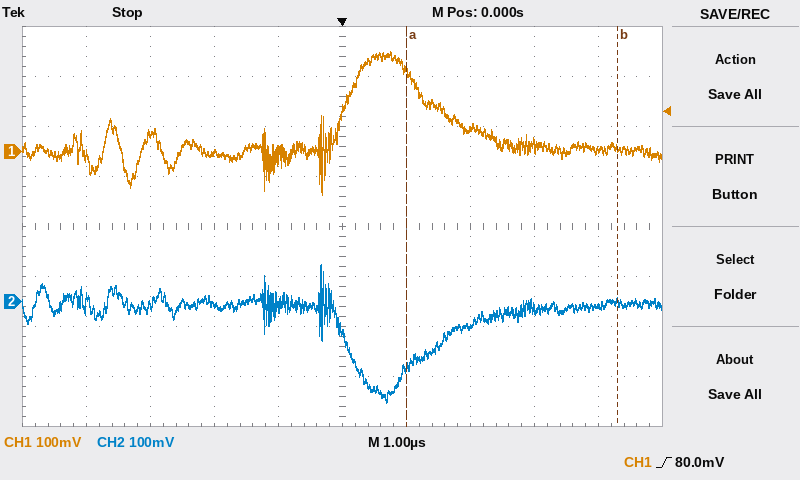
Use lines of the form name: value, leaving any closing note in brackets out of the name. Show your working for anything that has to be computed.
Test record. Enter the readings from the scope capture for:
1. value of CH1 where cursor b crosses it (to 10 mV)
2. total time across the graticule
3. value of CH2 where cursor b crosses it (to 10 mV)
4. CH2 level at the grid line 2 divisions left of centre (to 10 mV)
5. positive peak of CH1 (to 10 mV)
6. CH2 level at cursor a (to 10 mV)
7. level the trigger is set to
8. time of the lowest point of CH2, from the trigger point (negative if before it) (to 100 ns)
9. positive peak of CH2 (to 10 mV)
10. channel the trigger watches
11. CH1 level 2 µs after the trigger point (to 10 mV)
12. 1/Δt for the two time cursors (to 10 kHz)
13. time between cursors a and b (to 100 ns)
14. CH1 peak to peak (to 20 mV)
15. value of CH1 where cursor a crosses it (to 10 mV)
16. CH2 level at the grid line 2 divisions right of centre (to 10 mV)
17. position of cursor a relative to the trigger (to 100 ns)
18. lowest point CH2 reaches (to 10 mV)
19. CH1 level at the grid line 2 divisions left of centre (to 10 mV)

value of CH1 where cursor b crosses it: 10 mV
total time across the graticule: 10 µs
value of CH2 where cursor b crosses it: 0 mV
CH2 level at the grid line 2 divisions left of centre: -10 mV
positive peak of CH1: 200 mV
CH2 level at cursor a: -130 mV
level the trigger is set to: 80.0 mV
time of the lowest point of CH2, from the trigger point (negative if before it): +700 ns
positive peak of CH2: 70 mV
channel the trigger watches: CH1
CH1 level 2 µs after the trigger point: 50 mV
1/Δt for the two time cursors: 1 / 3.3 µs ≈ 300 kHz
time between cursors a and b: 3.3 µs
CH1 peak to peak: 280 mV
value of CH1 where cursor a crosses it: 160 mV
CH2 level at the grid line 2 divisions right of centre: -50 mV
position of cursor a relative to the trigger: +1.0 µs
lowest point CH2 reaches: -200 mV
CH1 level at the grid line 2 divisions left of centre: 0 mV
